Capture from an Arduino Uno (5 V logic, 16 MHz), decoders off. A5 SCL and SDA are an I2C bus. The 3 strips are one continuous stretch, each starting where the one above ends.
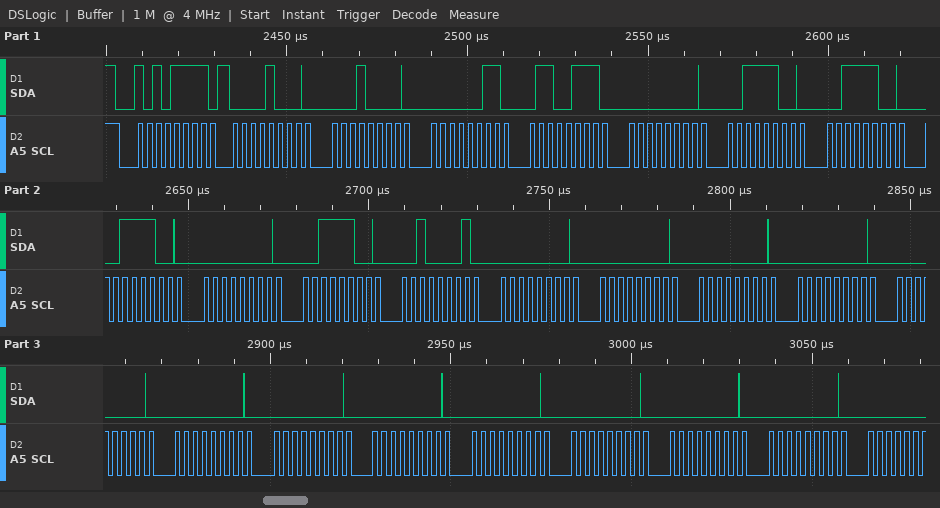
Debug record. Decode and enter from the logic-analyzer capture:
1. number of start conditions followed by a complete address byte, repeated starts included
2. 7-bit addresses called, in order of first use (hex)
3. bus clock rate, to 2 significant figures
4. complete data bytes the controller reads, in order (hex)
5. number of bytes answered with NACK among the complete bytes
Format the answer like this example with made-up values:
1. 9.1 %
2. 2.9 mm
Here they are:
1. 1
2. 0x57
3. 400 kHz
4. 08 10 03 67 00 3C 3C 3C 00 3C 21 00 00 00 00 00 00 00 00 00 00 00 00
5. 0
